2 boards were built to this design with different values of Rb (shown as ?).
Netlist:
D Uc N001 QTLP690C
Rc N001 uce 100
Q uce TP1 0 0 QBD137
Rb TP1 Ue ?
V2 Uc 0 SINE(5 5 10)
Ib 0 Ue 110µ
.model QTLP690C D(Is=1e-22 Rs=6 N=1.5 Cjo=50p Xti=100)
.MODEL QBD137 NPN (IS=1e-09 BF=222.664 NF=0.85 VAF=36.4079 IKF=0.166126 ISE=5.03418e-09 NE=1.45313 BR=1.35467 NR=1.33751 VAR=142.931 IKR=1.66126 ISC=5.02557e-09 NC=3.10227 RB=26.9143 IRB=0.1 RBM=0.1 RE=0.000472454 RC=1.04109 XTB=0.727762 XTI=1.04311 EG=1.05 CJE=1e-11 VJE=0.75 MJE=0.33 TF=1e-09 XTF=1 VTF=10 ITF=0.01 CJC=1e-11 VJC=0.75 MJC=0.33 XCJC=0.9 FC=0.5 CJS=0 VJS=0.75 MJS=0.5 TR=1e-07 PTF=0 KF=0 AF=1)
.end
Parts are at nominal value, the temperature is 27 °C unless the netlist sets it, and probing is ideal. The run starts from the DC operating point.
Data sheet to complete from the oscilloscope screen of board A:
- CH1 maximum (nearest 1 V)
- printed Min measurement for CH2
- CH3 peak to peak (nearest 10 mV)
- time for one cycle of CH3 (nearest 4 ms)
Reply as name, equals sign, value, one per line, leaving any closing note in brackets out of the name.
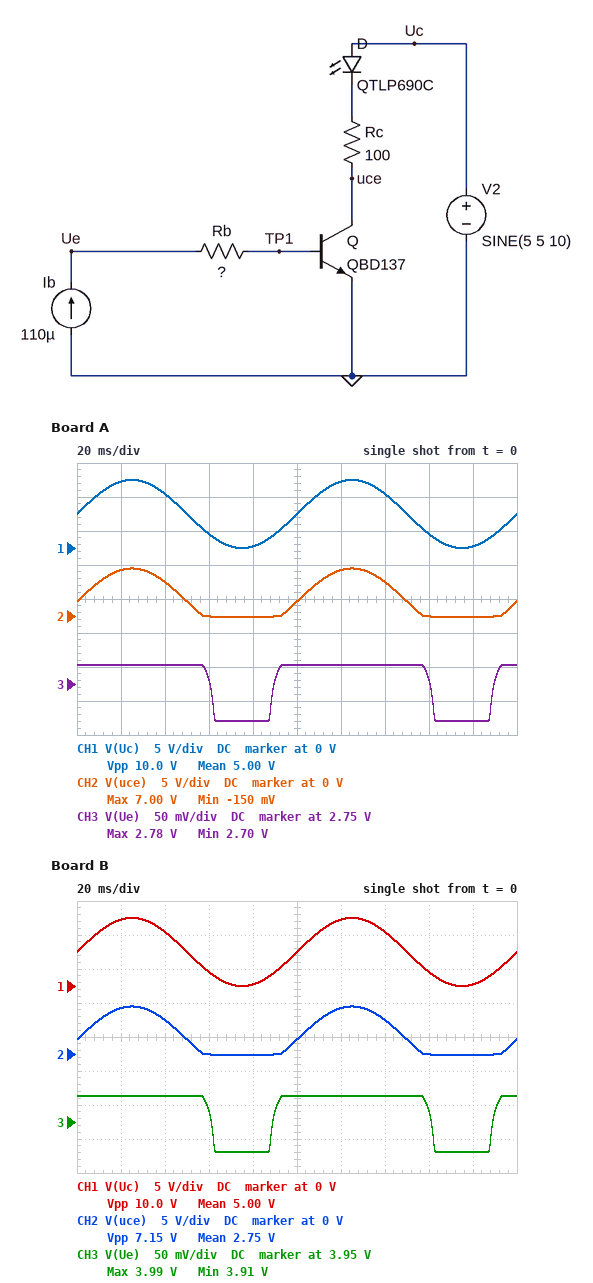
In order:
CH1 maximum = 10 V
printed Min measurement for CH2 = -150 mV
CH3 peak to peak = 80 mV
time for one cycle of CH3 = 100 ms
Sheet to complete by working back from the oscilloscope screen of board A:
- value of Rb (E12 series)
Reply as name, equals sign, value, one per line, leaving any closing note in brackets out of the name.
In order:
value of Rb = 22 kΩ
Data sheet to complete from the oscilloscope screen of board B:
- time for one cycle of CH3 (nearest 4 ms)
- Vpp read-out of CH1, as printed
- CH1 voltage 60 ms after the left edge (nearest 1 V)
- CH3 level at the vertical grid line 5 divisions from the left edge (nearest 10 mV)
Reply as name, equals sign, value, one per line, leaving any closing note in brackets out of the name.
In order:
time for one cycle of CH3 = 100 ms
Vpp read-out of CH1, as printed = 10.0 V
CH1 voltage 60 ms after the left edge = 2 V
CH3 level at the vertical grid line 5 divisions from the left edge = 3.99 V
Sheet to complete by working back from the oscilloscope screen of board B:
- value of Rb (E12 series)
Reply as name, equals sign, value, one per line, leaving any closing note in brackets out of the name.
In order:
value of Rb = 33 kΩ
